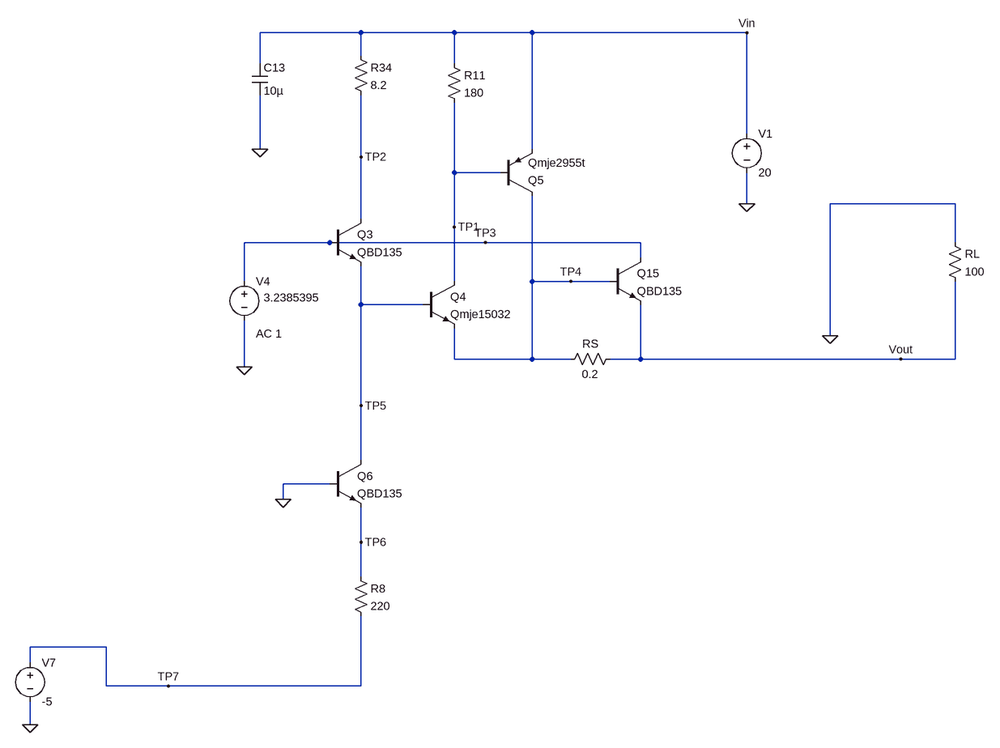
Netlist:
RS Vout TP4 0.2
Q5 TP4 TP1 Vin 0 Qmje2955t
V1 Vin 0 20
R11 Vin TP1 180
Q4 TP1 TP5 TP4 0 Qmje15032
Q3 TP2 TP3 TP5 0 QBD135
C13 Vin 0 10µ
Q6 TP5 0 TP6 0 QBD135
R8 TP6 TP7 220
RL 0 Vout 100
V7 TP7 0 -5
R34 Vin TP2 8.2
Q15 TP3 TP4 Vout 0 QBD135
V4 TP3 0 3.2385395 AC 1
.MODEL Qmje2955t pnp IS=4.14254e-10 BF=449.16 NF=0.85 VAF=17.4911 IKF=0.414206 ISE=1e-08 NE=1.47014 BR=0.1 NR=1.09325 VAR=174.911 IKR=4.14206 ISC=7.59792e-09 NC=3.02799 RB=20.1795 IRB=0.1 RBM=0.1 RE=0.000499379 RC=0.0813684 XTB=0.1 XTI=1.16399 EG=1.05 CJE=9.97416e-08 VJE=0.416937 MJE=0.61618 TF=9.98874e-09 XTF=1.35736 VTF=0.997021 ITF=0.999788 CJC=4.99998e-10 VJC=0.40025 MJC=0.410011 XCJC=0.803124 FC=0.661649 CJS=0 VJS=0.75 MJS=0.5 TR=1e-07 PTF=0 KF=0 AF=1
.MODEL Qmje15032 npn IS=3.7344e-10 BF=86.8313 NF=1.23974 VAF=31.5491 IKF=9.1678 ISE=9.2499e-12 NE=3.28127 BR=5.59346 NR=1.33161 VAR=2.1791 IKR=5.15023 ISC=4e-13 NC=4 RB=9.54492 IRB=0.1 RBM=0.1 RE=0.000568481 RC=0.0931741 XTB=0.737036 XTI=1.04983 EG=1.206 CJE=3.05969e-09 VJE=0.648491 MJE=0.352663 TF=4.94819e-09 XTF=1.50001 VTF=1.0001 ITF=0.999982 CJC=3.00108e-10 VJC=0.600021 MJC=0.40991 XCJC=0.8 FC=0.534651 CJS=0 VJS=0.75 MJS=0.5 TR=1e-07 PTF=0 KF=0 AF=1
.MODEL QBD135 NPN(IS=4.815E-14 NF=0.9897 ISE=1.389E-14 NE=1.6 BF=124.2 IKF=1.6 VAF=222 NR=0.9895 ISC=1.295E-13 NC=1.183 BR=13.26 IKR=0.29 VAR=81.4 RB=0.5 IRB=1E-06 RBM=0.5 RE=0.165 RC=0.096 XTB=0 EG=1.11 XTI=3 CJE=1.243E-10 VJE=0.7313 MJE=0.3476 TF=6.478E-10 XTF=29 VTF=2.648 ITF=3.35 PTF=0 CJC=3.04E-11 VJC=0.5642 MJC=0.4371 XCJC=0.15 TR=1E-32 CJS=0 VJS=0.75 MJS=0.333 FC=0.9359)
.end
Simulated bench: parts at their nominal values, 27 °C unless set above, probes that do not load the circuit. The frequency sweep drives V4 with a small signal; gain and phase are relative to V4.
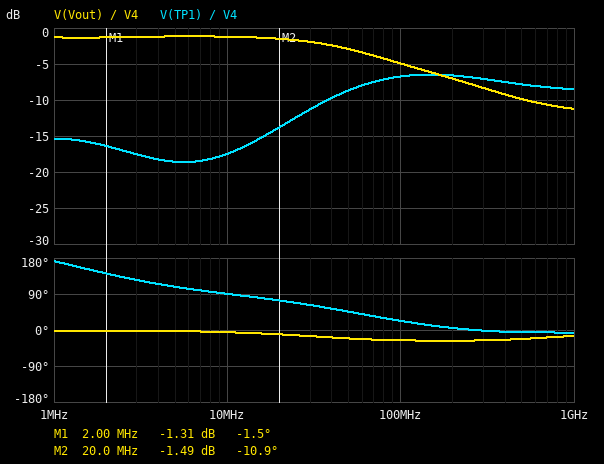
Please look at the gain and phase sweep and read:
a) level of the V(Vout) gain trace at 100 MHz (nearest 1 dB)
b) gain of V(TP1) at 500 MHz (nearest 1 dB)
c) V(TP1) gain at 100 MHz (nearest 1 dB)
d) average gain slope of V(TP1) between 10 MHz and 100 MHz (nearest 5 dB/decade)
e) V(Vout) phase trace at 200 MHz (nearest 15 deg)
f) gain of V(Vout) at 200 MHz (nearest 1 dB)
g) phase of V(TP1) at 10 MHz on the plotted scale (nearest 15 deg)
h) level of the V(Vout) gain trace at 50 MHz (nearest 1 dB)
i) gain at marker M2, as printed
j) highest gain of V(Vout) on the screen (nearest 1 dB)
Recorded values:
-5 dB
-8 dB
-7 dB
10 dB/decade
-30 deg
-7 dB
90 deg
-3 dB
-1.49 dB
-1 dB
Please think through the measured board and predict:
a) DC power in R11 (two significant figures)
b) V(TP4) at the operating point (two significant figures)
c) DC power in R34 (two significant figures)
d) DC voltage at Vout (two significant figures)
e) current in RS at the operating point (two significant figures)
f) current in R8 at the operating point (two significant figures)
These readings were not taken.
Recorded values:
790 µW
2.1 V
3.1 mW
2.1 V
21 mA
20 mA
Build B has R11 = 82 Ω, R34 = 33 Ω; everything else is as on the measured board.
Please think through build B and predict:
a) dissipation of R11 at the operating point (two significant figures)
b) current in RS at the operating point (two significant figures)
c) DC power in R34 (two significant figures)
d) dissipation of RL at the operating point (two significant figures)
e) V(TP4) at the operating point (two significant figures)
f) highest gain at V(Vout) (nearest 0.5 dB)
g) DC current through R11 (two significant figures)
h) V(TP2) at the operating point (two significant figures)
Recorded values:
1.7 mW
20 mA
12 mW
41 mW
2.0 V
0 dB
4.5 mA
19 V
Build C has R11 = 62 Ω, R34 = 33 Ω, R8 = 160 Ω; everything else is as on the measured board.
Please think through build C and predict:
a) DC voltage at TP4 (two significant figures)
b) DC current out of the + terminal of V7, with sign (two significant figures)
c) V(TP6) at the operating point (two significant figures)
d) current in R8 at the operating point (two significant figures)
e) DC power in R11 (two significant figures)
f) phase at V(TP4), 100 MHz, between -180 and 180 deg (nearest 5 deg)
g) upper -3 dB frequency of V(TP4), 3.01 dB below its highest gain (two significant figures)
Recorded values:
2.0 V
-27 mA
-700 mV
27 mA
2.2 mW
-30 deg
57 MHz
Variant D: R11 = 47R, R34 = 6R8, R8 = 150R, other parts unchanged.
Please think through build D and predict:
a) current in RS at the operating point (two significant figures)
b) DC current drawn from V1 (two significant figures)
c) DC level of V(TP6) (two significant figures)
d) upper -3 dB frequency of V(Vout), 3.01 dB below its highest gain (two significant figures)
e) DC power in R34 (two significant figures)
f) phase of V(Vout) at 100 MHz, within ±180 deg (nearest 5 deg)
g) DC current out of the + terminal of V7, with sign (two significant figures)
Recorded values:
20 mA
48 mA
-700 mV
58 MHz
5.4 mW
-30 deg
-29 mA
